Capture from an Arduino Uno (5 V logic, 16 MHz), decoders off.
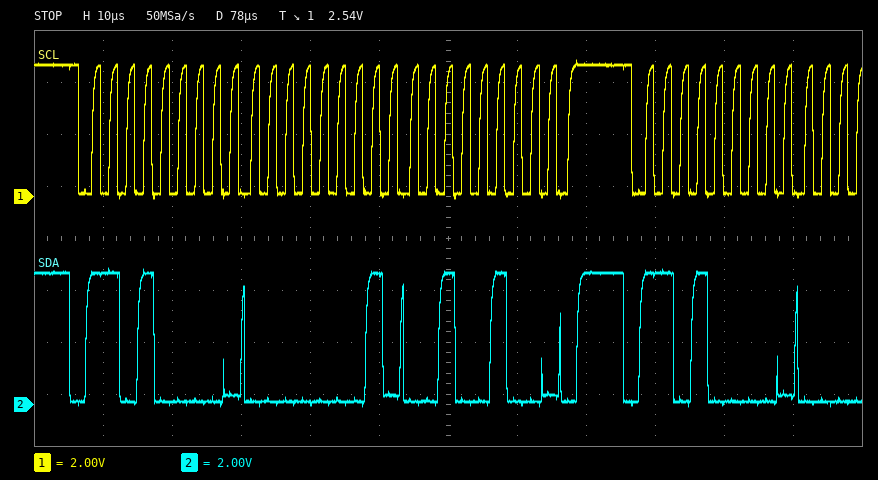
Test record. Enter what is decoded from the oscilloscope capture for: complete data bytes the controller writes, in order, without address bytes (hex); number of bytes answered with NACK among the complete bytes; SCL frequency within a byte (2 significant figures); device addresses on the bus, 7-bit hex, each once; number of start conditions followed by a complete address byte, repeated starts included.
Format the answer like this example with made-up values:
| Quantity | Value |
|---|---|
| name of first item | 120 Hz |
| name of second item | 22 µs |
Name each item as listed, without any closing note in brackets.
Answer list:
| Quantity | Value |
|---|---|
| complete data bytes the controller writes, in order, without address bytes | 01 24 |
| number of bytes answered with NACK among the complete bytes | 0 |
| SCL frequency within a byte | 400 kHz |
| device addresses on the bus, 7-bit hex, each once | 0x68 |
| number of start conditions followed by a complete address byte, repeated starts included | 2 |
